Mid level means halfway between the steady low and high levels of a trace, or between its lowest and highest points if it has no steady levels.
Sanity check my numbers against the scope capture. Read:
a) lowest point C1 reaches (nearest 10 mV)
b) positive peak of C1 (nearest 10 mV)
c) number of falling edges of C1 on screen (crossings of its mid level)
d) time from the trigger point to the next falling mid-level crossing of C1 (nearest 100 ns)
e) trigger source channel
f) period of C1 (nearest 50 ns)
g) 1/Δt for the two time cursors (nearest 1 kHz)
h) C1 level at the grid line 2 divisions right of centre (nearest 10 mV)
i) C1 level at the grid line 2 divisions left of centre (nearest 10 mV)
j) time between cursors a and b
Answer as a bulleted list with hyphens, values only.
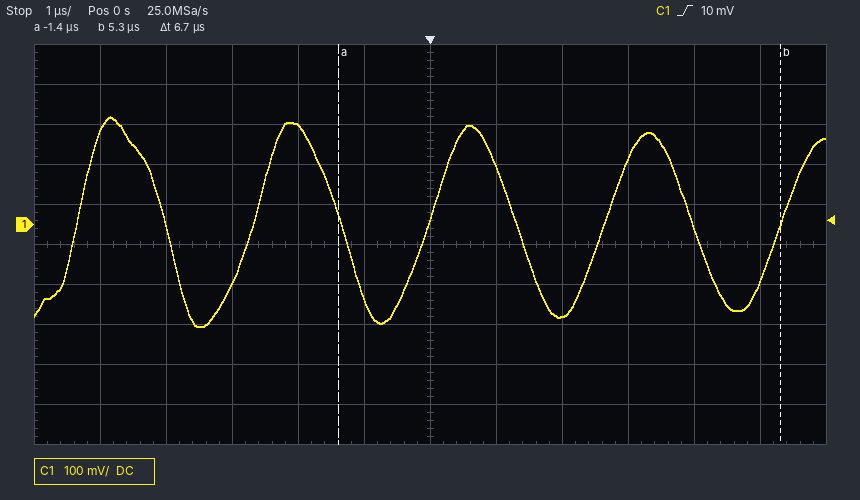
- -260 mV
- 270 mV
- 4
- 1.3 µs
- C1
- 2.65 µs
- 149 kHz
- -230 mV
- 250 mV
- 6.7 µs
